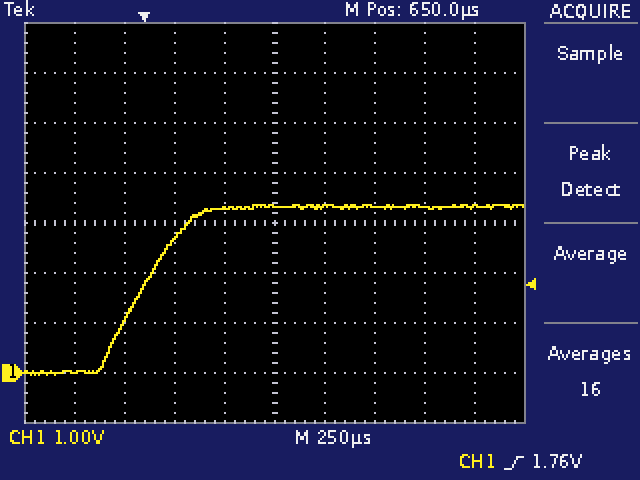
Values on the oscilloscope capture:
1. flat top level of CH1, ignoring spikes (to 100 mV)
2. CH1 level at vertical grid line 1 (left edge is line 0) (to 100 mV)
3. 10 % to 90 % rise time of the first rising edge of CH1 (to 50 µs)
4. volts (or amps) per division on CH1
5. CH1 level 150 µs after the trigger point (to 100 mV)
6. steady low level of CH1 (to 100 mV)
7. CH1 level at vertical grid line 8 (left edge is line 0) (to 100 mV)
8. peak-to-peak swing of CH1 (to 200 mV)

3.3 V
0.0 V
400 µs
1 V
2.7 V
0.0 V
3.3 V
3.4 V
